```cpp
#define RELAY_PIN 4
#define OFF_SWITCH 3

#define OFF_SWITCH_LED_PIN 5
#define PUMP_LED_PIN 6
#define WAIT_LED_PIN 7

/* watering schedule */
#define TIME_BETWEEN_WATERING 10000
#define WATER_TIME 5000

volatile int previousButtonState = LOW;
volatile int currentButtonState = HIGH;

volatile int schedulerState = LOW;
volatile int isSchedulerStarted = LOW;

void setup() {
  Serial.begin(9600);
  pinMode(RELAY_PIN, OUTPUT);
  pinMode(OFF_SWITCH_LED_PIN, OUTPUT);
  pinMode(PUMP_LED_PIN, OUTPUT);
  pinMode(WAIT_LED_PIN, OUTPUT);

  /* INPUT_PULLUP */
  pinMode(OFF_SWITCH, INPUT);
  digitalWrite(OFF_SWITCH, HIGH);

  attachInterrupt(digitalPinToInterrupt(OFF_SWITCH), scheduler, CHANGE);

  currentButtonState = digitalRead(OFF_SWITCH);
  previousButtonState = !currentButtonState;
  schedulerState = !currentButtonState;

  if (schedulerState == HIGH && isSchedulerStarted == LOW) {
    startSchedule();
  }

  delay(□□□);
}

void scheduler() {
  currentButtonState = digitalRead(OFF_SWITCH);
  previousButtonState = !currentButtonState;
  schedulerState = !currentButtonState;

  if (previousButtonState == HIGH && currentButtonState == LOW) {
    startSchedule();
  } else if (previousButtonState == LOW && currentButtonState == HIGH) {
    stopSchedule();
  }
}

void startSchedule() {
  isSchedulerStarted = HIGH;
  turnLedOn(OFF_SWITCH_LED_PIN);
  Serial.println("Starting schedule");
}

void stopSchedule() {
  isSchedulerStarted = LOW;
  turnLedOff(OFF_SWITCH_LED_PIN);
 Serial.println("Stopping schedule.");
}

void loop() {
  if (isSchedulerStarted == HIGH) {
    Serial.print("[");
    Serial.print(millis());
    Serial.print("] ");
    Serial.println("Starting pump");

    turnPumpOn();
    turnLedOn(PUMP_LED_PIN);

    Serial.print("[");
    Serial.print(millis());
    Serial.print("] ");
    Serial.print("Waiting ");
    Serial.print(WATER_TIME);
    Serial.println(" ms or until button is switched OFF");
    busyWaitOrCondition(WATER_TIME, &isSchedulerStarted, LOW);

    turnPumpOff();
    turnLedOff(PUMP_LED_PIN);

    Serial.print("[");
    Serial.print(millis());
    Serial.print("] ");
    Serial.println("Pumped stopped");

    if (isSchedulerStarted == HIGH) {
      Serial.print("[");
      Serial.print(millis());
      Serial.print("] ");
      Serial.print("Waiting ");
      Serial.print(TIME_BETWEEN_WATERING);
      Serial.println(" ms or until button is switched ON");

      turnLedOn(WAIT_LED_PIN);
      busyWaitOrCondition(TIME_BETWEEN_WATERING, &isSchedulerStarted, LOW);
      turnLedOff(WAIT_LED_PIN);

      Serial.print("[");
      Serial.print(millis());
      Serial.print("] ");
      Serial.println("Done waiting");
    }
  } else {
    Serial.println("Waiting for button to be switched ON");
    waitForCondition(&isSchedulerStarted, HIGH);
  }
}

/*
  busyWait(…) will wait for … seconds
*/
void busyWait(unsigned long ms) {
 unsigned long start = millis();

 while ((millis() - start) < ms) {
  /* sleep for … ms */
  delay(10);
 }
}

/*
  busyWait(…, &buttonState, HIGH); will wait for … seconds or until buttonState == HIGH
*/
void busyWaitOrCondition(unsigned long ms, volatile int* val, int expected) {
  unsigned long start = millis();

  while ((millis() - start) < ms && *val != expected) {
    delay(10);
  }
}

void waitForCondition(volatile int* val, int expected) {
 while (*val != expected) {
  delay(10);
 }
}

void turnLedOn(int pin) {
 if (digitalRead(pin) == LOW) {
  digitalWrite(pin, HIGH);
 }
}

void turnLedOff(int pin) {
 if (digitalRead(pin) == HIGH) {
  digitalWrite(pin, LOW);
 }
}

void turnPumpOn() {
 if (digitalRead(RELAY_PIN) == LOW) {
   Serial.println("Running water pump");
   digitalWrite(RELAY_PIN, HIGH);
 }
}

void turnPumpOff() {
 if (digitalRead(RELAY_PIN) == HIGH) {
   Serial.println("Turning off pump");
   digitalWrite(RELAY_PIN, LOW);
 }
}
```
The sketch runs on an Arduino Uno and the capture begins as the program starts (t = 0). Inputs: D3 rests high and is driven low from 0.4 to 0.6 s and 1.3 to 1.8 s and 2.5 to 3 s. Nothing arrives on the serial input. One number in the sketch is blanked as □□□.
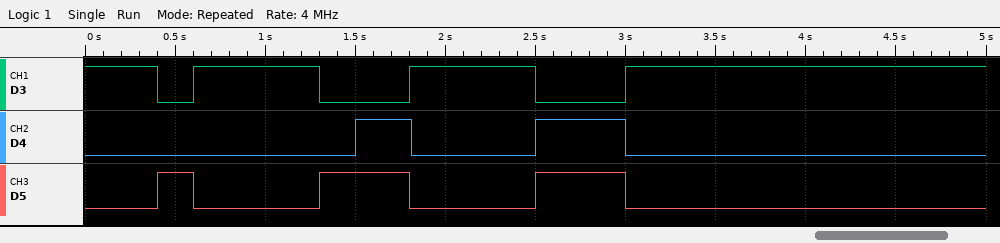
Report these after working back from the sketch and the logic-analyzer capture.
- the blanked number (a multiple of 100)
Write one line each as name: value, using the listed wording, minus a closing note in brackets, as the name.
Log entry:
the blanked number: 1500
